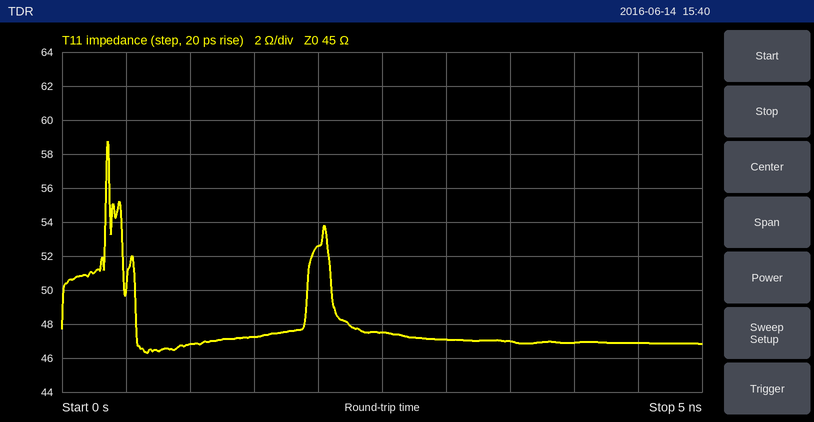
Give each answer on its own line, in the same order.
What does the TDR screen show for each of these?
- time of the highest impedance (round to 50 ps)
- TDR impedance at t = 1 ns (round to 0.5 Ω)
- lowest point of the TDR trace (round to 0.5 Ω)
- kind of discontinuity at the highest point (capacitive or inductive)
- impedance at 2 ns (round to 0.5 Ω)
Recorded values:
350 ps
47.0 Ω
46.5 Ω
inductive
52.5 Ω
